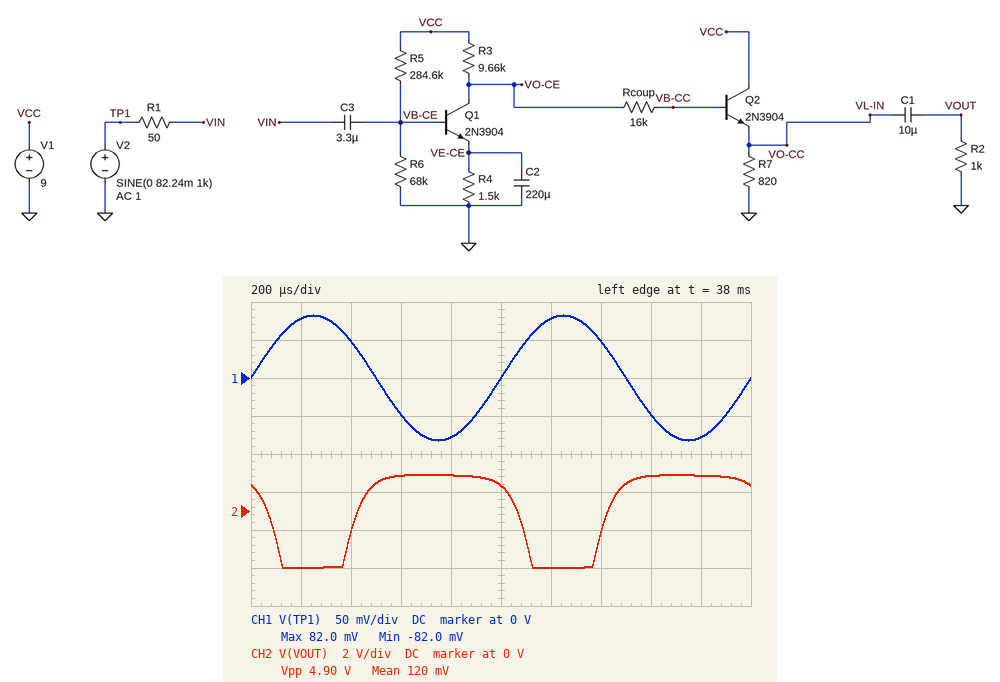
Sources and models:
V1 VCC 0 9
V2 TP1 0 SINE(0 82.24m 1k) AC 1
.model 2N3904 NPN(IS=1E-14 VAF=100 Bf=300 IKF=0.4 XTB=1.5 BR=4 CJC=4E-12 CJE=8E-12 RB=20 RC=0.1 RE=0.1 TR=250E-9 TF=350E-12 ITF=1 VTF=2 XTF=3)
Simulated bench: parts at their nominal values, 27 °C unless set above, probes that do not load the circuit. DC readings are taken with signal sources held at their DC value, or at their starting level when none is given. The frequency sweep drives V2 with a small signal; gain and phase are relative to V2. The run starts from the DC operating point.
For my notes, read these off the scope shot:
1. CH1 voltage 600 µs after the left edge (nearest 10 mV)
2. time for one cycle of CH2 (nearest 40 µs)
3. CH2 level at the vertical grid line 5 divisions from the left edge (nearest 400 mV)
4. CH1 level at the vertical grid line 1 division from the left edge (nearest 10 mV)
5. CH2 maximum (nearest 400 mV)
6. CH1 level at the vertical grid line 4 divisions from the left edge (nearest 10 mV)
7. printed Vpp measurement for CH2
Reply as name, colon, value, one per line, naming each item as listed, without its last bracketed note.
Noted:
CH1 voltage 600 µs after the left edge: -50 mV
time for one cycle of CH2: 1.00 ms
CH2 level at the vertical grid line 5 divisions from the left edge: 1.2 V
CH1 level at the vertical grid line 1 division from the left edge: 80 mV
CH2 maximum: 2.0 V
CH1 level at the vertical grid line 4 divisions from the left edge: -80 mV
printed Vpp measurement for CH2: 4.90 V
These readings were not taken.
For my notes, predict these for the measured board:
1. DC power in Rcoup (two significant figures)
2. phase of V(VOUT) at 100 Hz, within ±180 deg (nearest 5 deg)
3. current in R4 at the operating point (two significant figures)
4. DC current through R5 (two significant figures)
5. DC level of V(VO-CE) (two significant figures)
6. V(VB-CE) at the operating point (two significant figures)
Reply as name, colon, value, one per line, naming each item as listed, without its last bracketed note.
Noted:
DC power in Rcoup: 830 nW
phase of V(VOUT) at 100 Hz, within ±180 deg: -160 deg
current in R4 at the operating point: 650 µA
DC current through R5: 26 µA
DC level of V(VO-CE): 2.7 V
V(VB-CE) at the operating point: 1.6 V
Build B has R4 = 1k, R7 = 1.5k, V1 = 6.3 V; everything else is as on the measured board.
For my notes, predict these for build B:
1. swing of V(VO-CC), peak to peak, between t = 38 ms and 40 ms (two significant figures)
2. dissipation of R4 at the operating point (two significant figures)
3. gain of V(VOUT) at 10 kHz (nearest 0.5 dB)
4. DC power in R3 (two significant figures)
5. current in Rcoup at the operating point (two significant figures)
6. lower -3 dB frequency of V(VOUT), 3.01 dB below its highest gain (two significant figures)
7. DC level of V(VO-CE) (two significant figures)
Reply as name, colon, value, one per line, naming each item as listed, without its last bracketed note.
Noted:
swing of V(VO-CC), peak to peak, between t = 38 ms and 40 ms: 2.8 V
dissipation of R4 at the operating point: 240 µW
gain of V(VOUT) at 10 kHz: 43.0 dB
DC power in R3: 2.3 mW
current in Rcoup at the operating point: 1.9 µA
lower -3 dB frequency of V(VOUT), 3.01 dB below its highest gain: 24 Hz
DC level of V(VO-CE): 1.6 V
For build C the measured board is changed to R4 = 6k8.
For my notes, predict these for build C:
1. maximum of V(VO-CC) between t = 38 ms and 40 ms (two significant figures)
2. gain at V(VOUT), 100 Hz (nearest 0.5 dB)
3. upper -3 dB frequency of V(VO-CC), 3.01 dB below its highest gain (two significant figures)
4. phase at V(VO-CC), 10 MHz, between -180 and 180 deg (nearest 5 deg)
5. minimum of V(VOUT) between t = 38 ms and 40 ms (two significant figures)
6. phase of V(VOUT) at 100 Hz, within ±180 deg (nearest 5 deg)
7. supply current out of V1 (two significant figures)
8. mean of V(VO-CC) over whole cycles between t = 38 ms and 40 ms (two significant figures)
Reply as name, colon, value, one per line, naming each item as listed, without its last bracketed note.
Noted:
maximum of V(VO-CC) between t = 38 ms and 40 ms: 7.4 V
gain at V(VOUT), 100 Hz: 33.5 dB
upper -3 dB frequency of V(VO-CC), 3.01 dB below its highest gain: 1.8 MHz
phase at V(VO-CC), 10 MHz, between -180 and 180 deg: 55 deg
minimum of V(VOUT) between t = 38 ms and 40 ms: -3.3 V
phase of V(VOUT) at 100 Hz, within ±180 deg: -170 deg
supply current out of V1: 7.6 mA
mean of V(VO-CC) over whole cycles between t = 38 ms and 40 ms: 6.0 V
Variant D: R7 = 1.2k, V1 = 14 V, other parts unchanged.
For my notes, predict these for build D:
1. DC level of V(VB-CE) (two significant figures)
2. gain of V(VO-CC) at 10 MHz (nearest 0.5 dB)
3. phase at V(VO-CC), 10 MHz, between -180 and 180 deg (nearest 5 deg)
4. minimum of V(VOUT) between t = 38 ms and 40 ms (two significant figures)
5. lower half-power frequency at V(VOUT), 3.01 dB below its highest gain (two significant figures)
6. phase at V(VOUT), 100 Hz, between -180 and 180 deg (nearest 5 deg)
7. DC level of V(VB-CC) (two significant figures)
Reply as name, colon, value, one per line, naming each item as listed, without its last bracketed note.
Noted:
DC level of V(VB-CE): 2.5 V
gain of V(VO-CC) at 10 MHz: 22.0 dB
phase at V(VO-CC), 10 MHz, between -180 and 180 deg: 30 deg
minimum of V(VOUT) between t = 38 ms and 40 ms: -4.1 V
lower half-power frequency at V(VOUT), 3.01 dB below its highest gain: 43 Hz
phase at V(VOUT), 100 Hz, between -180 and 180 deg: -150 deg
DC level of V(VB-CC): 2.2 V
